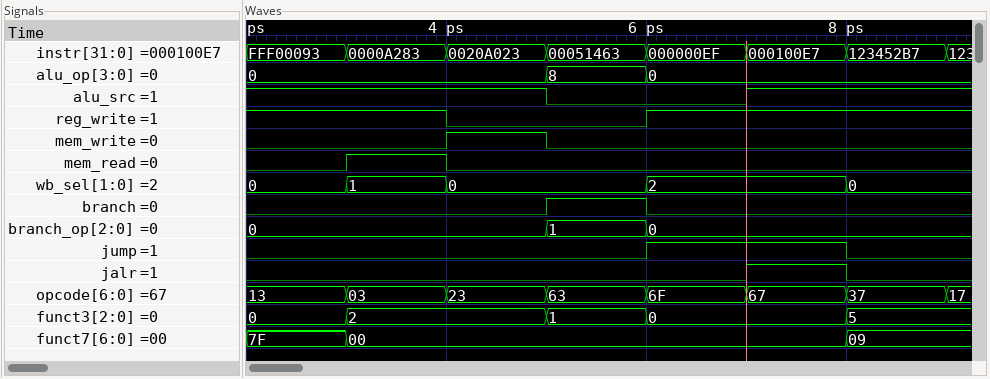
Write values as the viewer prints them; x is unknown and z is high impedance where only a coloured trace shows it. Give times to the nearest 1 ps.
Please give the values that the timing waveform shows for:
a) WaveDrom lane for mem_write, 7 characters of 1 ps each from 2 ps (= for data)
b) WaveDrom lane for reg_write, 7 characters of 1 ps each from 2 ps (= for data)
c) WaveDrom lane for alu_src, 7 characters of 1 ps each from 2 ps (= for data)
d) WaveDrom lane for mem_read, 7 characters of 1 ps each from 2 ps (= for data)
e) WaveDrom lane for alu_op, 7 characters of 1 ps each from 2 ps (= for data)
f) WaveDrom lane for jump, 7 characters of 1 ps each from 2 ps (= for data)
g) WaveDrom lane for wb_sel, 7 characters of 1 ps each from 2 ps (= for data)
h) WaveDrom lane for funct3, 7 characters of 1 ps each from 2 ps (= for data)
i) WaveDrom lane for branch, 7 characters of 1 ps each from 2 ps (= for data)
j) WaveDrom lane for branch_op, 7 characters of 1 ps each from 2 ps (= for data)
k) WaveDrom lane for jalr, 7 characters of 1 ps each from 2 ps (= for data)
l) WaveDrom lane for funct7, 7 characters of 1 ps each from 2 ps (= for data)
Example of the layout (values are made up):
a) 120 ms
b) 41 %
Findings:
a) {name: 'mem_write', wave: '0.10...'}
b) {name: 'reg_write', wave: '1.0.1..'}
c) {name: 'alu_src', wave: '1..0.1.'}
d) {name: 'mem_read', wave: '010....'}
e) {name: 'alu_op', wave: '=..==..', data: '0 8 0'}
f) {name: 'jump', wave: '0...1.0'}
g) {name: 'wb_sel', wave: '===.=.=', data: '0 1 0 2 0'}
h) {name: 'funct3', wave: '==.==.=', data: '0 2 1 0 5'}
i) {name: 'branch', wave: '0..10..'}
j) {name: 'branch_op', wave: '=..==..', data: '0 1 0'}
k) {name: 'jalr', wave: '0....10'}
l) {name: 'funct7', wave: '==....=', data: '7F 00 09'}
